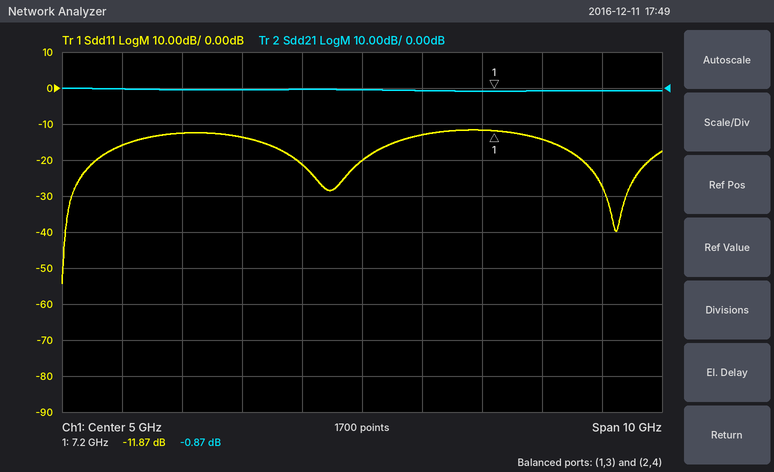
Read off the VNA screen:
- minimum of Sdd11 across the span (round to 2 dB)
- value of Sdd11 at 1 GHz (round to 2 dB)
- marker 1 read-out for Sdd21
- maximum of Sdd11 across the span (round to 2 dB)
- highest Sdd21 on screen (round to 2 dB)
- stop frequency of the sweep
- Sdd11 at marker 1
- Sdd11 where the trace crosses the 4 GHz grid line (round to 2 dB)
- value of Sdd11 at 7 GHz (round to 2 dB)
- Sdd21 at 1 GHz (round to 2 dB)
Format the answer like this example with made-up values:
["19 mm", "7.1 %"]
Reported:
["-54 dB", "-16 dB", "-0.87 dB", "-12 dB", "0 dB", "10 GHz", "-11.87 dB", "-22 dB", "-12 dB", "0 dB"]
